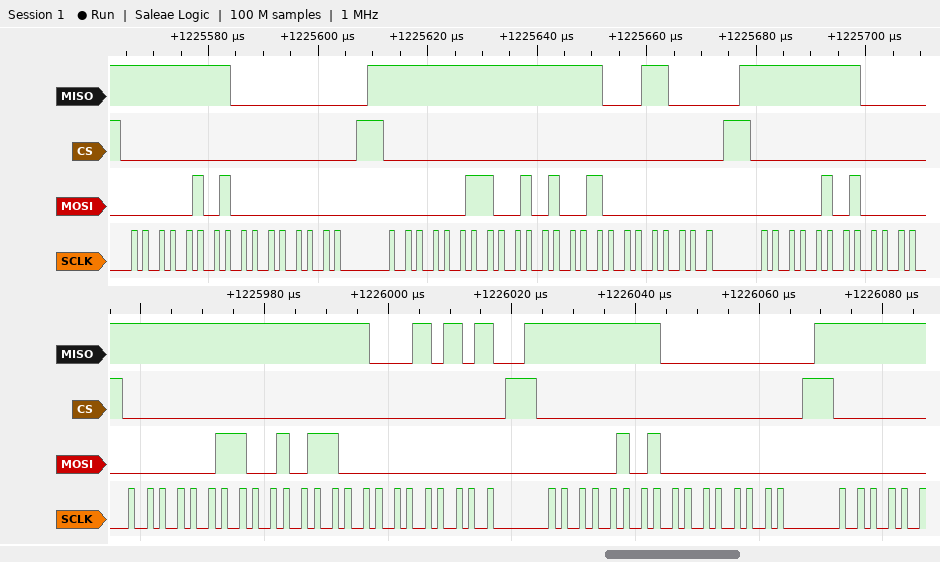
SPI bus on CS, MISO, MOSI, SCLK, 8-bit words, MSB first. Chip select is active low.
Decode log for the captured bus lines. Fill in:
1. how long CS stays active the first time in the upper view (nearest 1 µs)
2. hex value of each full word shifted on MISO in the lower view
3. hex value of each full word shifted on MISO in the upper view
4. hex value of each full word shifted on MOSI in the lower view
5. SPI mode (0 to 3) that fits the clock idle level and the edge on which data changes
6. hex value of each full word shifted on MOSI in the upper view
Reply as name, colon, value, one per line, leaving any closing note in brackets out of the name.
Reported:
how long CS stays active the first time in the upper view: 43 µs
hex value of each full word shifted on MISO in the lower view: FF, FF, 15, FF, 00
hex value of each full word shifted on MISO in the upper view: FF, 00, FF, FF, 18, FF
hex value of each full word shifted on MOSI in the lower view: 03, 2C, 00, 05, 00
SPI mode (0 to 3) that fits the clock idle level and the edge on which data changes: 0
hex value of each full word shifted on MOSI in the upper view: 05, 00, 03, 29, 00, 05
